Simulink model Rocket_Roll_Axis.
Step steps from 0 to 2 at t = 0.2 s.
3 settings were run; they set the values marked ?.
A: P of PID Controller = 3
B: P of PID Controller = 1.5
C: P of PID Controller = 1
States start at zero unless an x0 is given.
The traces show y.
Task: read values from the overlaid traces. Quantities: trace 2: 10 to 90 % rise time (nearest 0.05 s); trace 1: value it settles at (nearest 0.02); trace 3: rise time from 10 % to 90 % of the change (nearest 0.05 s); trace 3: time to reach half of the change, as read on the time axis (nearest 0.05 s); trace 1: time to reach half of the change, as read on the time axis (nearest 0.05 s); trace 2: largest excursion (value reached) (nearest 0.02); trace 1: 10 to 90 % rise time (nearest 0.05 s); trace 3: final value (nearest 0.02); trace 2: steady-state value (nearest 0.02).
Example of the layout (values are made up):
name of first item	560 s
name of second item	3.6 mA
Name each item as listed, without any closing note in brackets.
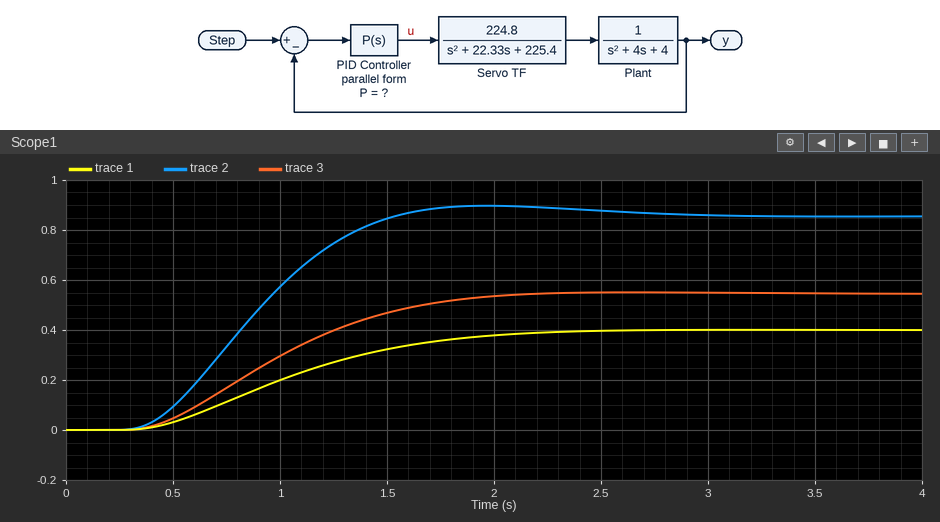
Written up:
trace 2: 10 to 90 % rise time	0.80 s
trace 1: value it settles at	0.40
trace 3: rise time from 10 % to 90 % of the change	1.10 s
trace 3: time to reach half of the change, as read on the time axis	0.95 s
trace 1: time to reach half of the change, as read on the time axis	1.00 s
trace 2: largest excursion (value reached)	0.90
trace 1: 10 to 90 % rise time	1.25 s
trace 3: final value	0.54
trace 2: steady-state value	0.86
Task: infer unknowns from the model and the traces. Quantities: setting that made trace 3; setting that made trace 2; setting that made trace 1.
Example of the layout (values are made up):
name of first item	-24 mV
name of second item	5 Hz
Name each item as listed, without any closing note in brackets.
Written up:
setting that made trace 3	B
setting that made trace 2	A
setting that made trace 1	C
